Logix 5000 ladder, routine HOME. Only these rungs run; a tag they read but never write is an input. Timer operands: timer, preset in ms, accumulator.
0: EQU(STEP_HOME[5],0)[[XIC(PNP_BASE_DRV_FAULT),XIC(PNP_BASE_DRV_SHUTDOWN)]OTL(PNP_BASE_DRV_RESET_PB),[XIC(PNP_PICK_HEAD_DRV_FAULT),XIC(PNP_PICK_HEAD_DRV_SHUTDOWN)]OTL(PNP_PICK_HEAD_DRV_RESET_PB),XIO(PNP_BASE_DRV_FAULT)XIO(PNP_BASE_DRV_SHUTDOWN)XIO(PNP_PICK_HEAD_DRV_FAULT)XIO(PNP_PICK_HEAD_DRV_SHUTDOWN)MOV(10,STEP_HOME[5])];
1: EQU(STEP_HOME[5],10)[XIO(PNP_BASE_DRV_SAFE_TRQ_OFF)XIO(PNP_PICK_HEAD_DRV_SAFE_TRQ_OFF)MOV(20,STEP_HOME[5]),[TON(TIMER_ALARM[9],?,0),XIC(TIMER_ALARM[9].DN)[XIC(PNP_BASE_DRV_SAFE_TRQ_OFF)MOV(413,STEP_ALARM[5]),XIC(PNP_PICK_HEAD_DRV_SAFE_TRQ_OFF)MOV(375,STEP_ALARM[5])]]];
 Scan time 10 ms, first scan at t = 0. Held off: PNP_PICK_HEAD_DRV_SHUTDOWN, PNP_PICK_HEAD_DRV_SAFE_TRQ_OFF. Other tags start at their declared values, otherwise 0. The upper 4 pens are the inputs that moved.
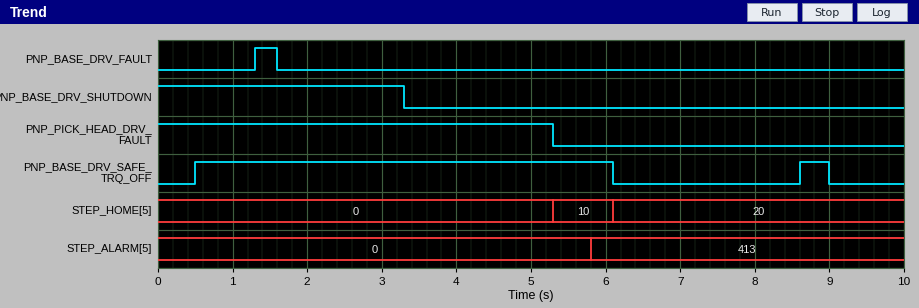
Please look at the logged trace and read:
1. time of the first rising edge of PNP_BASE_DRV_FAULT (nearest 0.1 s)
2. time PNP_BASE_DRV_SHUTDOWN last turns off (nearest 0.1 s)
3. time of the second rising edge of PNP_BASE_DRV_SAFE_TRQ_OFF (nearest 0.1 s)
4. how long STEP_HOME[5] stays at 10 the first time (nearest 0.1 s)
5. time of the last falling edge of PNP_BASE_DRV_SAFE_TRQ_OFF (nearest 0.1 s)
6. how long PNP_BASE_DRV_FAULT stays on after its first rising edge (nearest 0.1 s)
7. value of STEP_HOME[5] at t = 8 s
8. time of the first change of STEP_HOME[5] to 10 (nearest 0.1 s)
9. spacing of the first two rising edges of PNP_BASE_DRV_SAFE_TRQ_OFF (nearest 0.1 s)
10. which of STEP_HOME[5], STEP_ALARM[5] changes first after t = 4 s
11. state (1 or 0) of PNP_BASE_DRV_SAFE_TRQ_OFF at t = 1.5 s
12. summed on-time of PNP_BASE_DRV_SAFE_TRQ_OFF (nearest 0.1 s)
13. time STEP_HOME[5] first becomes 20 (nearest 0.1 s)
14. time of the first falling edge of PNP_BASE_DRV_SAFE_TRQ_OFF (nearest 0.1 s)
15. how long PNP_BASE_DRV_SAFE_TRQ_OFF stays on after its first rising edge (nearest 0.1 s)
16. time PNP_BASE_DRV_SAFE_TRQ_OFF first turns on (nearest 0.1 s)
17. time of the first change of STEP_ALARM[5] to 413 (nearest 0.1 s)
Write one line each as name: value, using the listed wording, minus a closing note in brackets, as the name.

time of the first rising edge of PNP_BASE_DRV_FAULT: 1.3 s
time PNP_BASE_DRV_SHUTDOWN last turns off: 3.3 s
time of the second rising edge of PNP_BASE_DRV_SAFE_TRQ_OFF: 8.6 s
how long STEP_HOME[5] stays at 10 the first time: 0.8 s
time of the last falling edge of PNP_BASE_DRV_SAFE_TRQ_OFF: 9.0 s
how long PNP_BASE_DRV_FAULT stays on after its first rising edge: 0.3 s
value of STEP_HOME[5] at t = 8 s: 20
time of the first change of STEP_HOME[5] to 10: 5.3 s
spacing of the first two rising edges of PNP_BASE_DRV_SAFE_TRQ_OFF: 8.1 s
which of STEP_HOME[5], STEP_ALARM[5] changes first after t = 4 s: STEP_HOME[5]
state (1 or 0) of PNP_BASE_DRV_SAFE_TRQ_OFF at t = 1.5 s: 1
summed on-time of PNP_BASE_DRV_SAFE_TRQ_OFF: 6.0 s
time STEP_HOME[5] first becomes 20: 6.1 s
time of the first falling edge of PNP_BASE_DRV_SAFE_TRQ_OFF: 6.1 s
how long PNP_BASE_DRV_SAFE_TRQ_OFF stays on after its first rising edge: 5.6 s
time PNP_BASE_DRV_SAFE_TRQ_OFF first turns on: 0.5 s
time of the first change of STEP_ALARM[5] to 413: 5.8 s
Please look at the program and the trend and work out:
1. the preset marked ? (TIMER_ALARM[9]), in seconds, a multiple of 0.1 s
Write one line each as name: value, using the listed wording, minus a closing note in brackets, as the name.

the preset marked ? (TIMER_ALARM[9]), in seconds, a multiple of 0.1 s: 0.5 s
